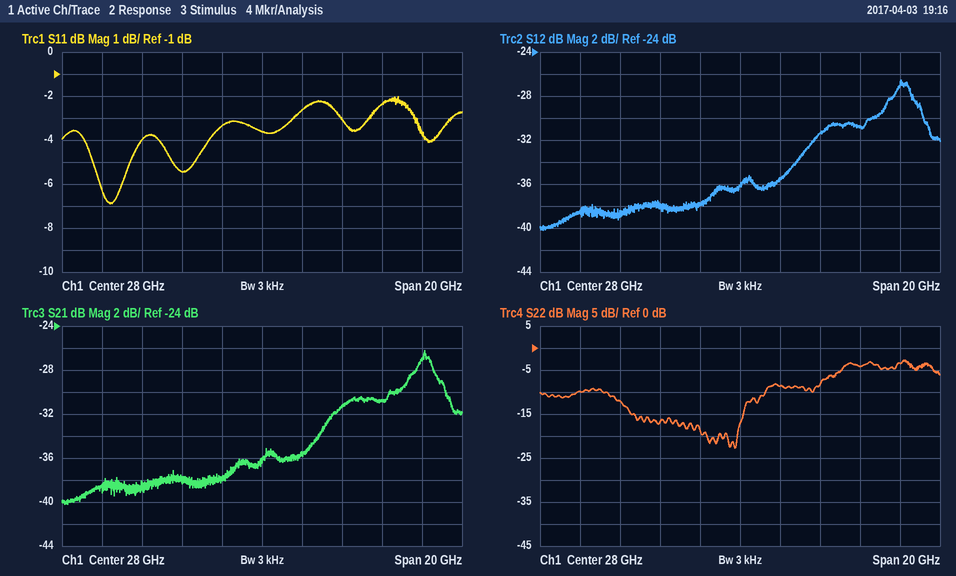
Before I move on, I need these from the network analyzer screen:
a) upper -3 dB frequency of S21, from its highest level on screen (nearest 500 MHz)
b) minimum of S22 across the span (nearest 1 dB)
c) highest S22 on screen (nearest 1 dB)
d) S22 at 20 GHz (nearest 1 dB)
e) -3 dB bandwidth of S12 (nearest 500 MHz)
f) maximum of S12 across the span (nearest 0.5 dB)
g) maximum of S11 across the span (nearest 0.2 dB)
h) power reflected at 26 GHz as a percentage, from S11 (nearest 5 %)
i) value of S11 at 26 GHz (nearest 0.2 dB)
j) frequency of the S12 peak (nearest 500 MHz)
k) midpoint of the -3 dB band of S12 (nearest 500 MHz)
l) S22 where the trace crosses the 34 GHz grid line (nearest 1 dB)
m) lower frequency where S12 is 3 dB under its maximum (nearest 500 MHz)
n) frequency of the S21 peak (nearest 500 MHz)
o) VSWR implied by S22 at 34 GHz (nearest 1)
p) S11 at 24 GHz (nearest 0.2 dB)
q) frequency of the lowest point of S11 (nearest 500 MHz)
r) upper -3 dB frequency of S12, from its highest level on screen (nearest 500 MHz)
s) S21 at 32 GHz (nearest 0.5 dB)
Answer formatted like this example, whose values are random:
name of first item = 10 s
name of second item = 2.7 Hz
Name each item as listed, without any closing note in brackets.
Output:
upper -3 dB frequency of S21, from its highest level on screen = 37.0 GHz
minimum of S22 across the span = -23 dB
highest S22 on screen = -3 dB
S22 at 20 GHz = -10 dB
-3 dB bandwidth of S12 = 2.0 GHz
maximum of S12 across the span = -26.5 dB
maximum of S11 across the span = -2.0 dB
power reflected at 26 GHz as a percentage, from S11 = 45 %
value of S11 at 26 GHz = -3.4 dB
frequency of the S12 peak = 36.0 GHz
midpoint of the -3 dB band of S12 = 36.0 GHz
S22 where the trace crosses the 34 GHz grid line = -4 dB
lower frequency where S12 is 3 dB under its maximum = 35.0 GHz
frequency of the S21 peak = 36.0 GHz
VSWR implied by S22 at 34 GHz = 4
S11 at 24 GHz = -5.4 dB
frequency of the lowest point of S11 = 20.5 GHz
upper -3 dB frequency of S12, from its highest level on screen = 37.0 GHz
S21 at 32 GHz = -31.5 dB
